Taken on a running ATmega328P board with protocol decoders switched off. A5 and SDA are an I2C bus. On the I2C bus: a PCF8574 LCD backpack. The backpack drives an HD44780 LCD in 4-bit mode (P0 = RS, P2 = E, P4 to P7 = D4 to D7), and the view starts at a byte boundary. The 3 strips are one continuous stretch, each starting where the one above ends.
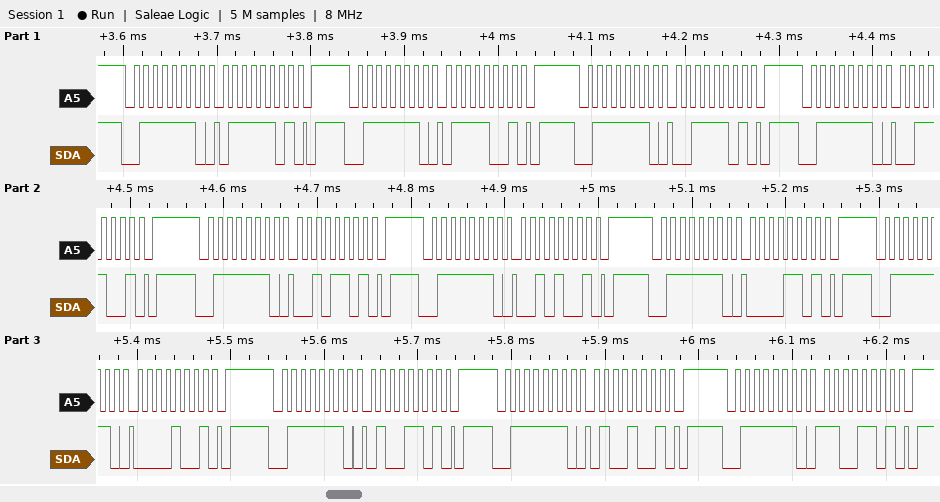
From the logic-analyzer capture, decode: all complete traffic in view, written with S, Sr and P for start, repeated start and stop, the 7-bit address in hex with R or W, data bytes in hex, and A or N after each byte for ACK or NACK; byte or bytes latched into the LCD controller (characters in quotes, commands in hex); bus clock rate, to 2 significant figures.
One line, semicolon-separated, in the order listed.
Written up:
S 3FW A 7D A P S 3FW A 79 A P S 3FW A 3D A P S 3FW A 39 A P S 3FW A 2D A P S 3FW A 29 A P S 3FW A 0D A P S 3FW A 09 A P S 3FW A 4D A P S 3FW A 49 A P S 3FW A CD A P; 's' ' '; 100 kHz
